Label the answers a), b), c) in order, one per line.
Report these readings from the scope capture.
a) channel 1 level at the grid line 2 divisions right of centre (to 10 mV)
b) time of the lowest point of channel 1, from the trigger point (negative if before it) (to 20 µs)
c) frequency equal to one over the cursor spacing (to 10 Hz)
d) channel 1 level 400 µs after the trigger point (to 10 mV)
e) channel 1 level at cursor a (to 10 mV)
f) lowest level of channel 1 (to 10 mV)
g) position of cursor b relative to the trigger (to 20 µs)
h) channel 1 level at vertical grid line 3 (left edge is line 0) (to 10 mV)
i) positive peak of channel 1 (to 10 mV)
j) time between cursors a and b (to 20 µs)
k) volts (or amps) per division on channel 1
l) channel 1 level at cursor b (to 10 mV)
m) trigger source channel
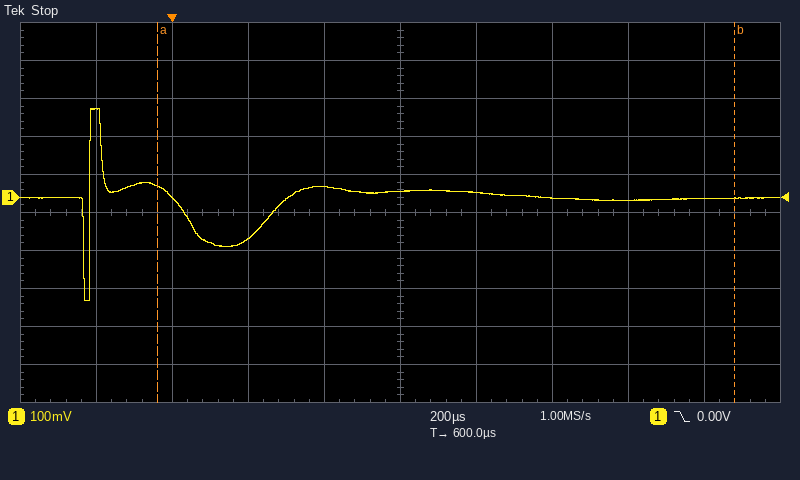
a) 0 mV
b) -220 µs
c) 660 Hz
d) 30 mV
e) 30 mV
f) -270 mV
g) +1.48 ms
h) -110 mV
i) 230 mV
j) 1.52 ms
k) 100 mV
l) 0 mV
m) channel 1
